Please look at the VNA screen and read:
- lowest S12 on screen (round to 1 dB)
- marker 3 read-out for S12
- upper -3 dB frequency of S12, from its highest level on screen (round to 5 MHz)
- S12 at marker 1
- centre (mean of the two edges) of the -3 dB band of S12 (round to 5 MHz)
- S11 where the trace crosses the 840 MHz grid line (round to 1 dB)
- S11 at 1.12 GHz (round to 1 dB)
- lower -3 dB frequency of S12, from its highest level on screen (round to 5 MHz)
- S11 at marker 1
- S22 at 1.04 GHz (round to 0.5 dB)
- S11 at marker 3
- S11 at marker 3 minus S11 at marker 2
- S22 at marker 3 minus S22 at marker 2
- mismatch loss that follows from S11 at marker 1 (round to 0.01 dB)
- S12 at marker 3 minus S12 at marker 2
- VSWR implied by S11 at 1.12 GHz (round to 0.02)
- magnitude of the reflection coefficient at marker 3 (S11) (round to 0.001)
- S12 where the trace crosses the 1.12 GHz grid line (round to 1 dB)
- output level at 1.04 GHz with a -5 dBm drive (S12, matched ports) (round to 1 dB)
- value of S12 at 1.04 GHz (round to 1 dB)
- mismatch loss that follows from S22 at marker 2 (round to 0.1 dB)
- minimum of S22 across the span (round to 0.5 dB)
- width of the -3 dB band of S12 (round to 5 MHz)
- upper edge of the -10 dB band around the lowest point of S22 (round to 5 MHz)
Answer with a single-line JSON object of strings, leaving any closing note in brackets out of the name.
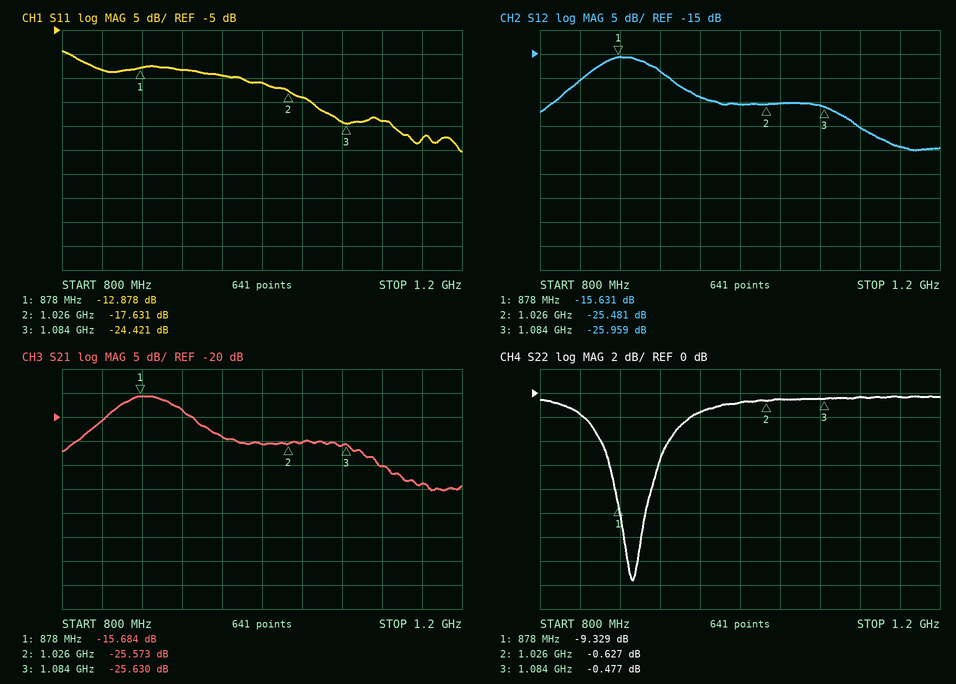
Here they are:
{"lowest S12 on screen": "-35 dB", "marker 3 read-out for S12": "-25.959 dB", "upper -3 dB frequency of S12, from its highest level on screen": "920 MHz", "S12 at marker 1": "-15.631 dB", "centre (mean of the two edges) of the -3 dB band of S12": "885 MHz", "S11 where the trace crosses the 840 MHz grid line": "-13 dB", "S11 at 1.12 GHz": "-24 dB", "lower -3 dB frequency of S12, from its highest level on screen": "850 MHz", "S11 at marker 1": "-12.878 dB", "S22 at 1.04 GHz": "-0.5 dB", "S11 at marker 3": "-24.421 dB", "S11 at marker 3 minus S11 at marker 2": "-6.790 dB", "S22 at marker 3 minus S22 at marker 2": "0.150 dB", "mismatch loss that follows from S11 at marker 1": "0.23 dB", "S12 at marker 3 minus S12 at marker 2": "-0.478 dB", "VSWR implied by S11 at 1.12 GHz": "1.14", "magnitude of the reflection coefficient at marker 3 (S11)": "0.060", "S12 where the trace crosses the 1.12 GHz grid line": "-30 dB", "output level at 1.04 GHz with a -5 dBm drive (S12, matched ports)": "-30 dBm", "value of S12 at 1.04 GHz": "-25 dB", "mismatch loss that follows from S22 at marker 2": "8.7 dB", "minimum of S22 across the span": "-15.5 dB", "width of the -3 dB band of S12": "70 MHz", "upper edge of the -10 dB band around the lowest point of S22": "905 MHz"}
